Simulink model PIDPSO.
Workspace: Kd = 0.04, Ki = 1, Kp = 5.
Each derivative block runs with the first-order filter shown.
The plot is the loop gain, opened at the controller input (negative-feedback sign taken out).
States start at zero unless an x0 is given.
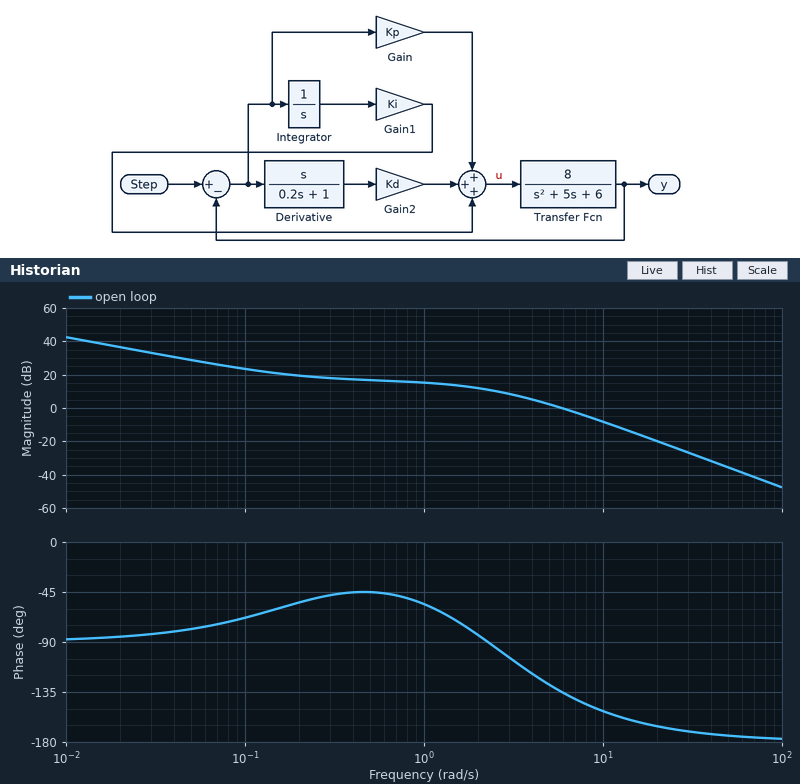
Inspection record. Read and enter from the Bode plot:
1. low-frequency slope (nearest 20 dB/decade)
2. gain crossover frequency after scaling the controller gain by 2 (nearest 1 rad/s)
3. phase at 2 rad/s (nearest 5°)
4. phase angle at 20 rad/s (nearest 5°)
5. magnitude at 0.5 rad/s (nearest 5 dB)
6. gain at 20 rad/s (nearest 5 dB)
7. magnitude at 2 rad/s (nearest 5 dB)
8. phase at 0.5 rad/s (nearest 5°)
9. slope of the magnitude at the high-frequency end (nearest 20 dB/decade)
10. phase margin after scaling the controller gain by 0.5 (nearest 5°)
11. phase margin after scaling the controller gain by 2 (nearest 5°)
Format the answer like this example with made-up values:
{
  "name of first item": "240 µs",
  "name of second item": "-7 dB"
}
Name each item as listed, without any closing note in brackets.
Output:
{
  "low-frequency slope": "-20 dB/decade",
  "gain crossover frequency after scaling the controller gain by 2": "9 rad/s",
  "phase at 2 rad/s": "-85°",
  "phase angle at 20 rad/s": "-165°",
  "magnitude at 0.5 rad/s": "15 dB",
  "gain at 20 rad/s": "-20 dB",
  "magnitude at 2 rad/s": "10 dB",
  "phase at 0.5 rad/s": "-45°",
  "slope of the magnitude at the high-frequency end": "-40 dB/decade",
  "phase margin after scaling the controller gain by 0.5": "65°",
  "phase margin after scaling the controller gain by 2": "30°"
}
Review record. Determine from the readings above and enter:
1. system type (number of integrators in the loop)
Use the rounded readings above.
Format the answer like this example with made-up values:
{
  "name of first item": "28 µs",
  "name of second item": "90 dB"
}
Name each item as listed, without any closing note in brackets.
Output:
{
  "system type": "1"
}
